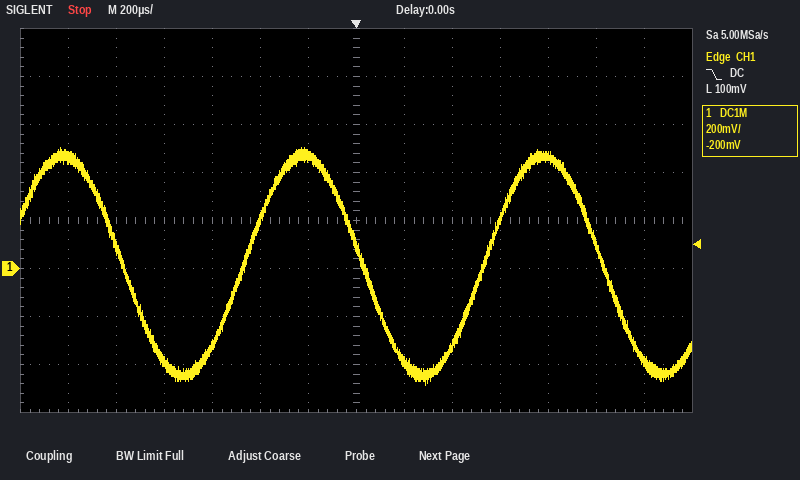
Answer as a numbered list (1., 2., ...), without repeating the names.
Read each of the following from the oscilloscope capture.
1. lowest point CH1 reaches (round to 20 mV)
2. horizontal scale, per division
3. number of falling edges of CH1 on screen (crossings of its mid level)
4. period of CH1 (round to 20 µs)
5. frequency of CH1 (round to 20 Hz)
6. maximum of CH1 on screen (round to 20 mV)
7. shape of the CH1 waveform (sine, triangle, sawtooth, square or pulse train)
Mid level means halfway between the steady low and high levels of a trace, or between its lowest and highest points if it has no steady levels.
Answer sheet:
1. -480 mV
2. 200 µs
3. 3
4. 1.00 ms
5. 1.00 kHz
6. 500 mV
7. sine
